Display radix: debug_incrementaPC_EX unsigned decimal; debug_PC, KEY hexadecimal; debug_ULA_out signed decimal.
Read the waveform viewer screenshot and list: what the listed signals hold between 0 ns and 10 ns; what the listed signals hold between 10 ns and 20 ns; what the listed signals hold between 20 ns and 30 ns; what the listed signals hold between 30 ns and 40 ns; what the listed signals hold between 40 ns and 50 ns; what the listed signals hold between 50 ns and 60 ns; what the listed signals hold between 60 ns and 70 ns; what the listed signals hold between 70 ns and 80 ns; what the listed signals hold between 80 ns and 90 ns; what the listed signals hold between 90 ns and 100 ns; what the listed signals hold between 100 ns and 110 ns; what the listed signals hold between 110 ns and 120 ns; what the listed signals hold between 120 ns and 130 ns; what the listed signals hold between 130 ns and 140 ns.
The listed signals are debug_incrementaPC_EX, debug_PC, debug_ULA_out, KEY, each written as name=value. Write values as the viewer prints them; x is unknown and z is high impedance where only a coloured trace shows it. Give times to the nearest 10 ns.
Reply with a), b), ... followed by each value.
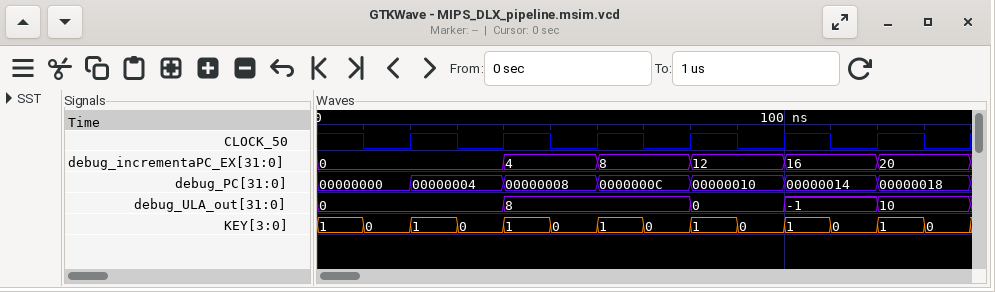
a) debug_incrementaPC_EX=0, debug_PC=00000000, debug_ULA_out=0, KEY=1
b) debug_incrementaPC_EX=0, debug_PC=00000000, debug_ULA_out=0, KEY=0
c) debug_incrementaPC_EX=0, debug_PC=00000004, debug_ULA_out=0, KEY=1
d) debug_incrementaPC_EX=0, debug_PC=00000004, debug_ULA_out=0, KEY=0
e) debug_incrementaPC_EX=4, debug_PC=00000008, debug_ULA_out=8, KEY=1
f) debug_incrementaPC_EX=4, debug_PC=00000008, debug_ULA_out=8, KEY=0
g) debug_incrementaPC_EX=8, debug_PC=0000000C, debug_ULA_out=8, KEY=1
h) debug_incrementaPC_EX=8, debug_PC=0000000C, debug_ULA_out=8, KEY=0
i) debug_incrementaPC_EX=12, debug_PC=00000010, debug_ULA_out=0, KEY=1
j) debug_incrementaPC_EX=12, debug_PC=00000010, debug_ULA_out=0, KEY=0
k) debug_incrementaPC_EX=16, debug_PC=00000014, debug_ULA_out=-1, KEY=1
l) debug_incrementaPC_EX=16, debug_PC=00000014, debug_ULA_out=-1, KEY=0
m) debug_incrementaPC_EX=20, debug_PC=00000018, debug_ULA_out=10, KEY=1
n) debug_incrementaPC_EX=20, debug_PC=00000018, debug_ULA_out=10, KEY=0
